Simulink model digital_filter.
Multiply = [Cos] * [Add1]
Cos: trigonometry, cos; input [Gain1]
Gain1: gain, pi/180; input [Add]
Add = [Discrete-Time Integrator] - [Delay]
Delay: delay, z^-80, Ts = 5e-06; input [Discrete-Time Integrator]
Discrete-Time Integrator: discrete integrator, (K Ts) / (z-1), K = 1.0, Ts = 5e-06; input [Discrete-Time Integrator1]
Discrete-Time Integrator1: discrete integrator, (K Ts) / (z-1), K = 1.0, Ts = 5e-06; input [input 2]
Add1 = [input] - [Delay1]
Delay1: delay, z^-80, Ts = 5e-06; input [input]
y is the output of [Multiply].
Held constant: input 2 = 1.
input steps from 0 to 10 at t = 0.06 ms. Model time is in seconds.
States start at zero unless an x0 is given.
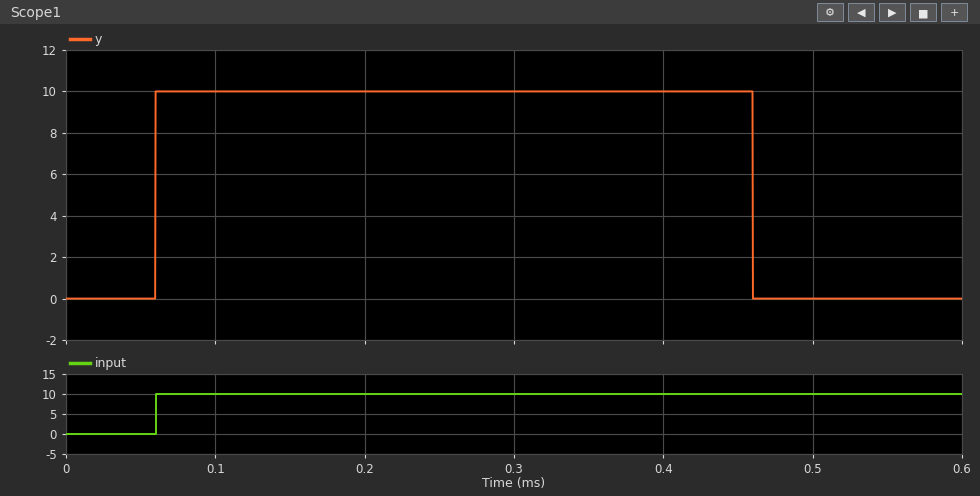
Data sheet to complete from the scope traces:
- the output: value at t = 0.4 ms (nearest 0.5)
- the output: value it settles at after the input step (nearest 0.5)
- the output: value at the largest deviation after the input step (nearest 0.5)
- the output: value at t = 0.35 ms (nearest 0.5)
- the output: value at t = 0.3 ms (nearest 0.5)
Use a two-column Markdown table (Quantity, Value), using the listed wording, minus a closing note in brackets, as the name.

| Quantity | Value |
|---|---|
| the output: value at t = 0.4 ms | 10.0 |
| the output: value it settles at after the input step | 0.0 |
| the output: value at the largest deviation after the input step | 10.0 |
| the output: value at t = 0.35 ms | 10.0 |
| the output: value at t = 0.3 ms | 10.0 |
